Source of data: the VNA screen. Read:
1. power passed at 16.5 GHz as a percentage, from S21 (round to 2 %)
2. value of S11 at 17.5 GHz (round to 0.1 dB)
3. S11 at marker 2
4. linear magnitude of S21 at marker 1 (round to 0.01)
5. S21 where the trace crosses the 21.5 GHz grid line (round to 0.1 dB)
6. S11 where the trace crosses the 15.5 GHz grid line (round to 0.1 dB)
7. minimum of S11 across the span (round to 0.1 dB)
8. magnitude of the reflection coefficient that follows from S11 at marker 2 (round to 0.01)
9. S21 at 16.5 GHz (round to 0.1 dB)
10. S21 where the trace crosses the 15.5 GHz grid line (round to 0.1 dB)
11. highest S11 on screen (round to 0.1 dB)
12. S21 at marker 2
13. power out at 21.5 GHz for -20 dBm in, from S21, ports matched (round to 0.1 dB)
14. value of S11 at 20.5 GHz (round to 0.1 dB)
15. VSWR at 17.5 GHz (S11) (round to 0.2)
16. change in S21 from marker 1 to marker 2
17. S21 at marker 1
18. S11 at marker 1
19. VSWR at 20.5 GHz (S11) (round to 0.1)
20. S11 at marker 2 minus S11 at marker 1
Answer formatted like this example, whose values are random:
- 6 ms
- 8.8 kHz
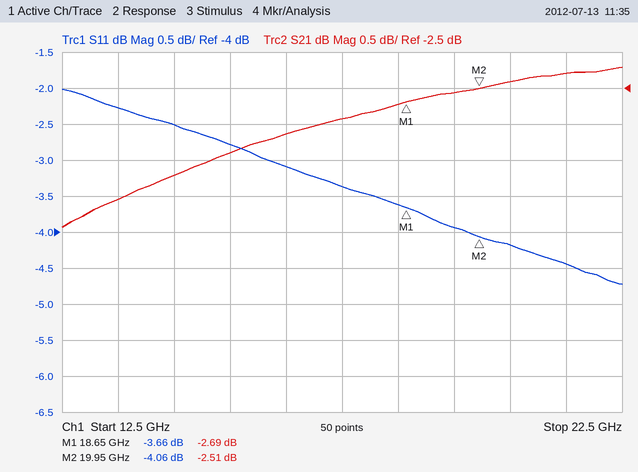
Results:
- 48 %
- -3.4 dB
- -4.06 dB
- 0.73
- -2.3 dB
- -2.8 dB
- -4.7 dB
- 0.63
- -3.1 dB
- -3.4 dB
- -2.0 dB
- -2.51 dB
- -22.3 dBm
- -4.2 dB
- 5.2
- 0.18 dB
- -2.69 dB
- -3.66 dB
- 4.2
- -0.40 dB
